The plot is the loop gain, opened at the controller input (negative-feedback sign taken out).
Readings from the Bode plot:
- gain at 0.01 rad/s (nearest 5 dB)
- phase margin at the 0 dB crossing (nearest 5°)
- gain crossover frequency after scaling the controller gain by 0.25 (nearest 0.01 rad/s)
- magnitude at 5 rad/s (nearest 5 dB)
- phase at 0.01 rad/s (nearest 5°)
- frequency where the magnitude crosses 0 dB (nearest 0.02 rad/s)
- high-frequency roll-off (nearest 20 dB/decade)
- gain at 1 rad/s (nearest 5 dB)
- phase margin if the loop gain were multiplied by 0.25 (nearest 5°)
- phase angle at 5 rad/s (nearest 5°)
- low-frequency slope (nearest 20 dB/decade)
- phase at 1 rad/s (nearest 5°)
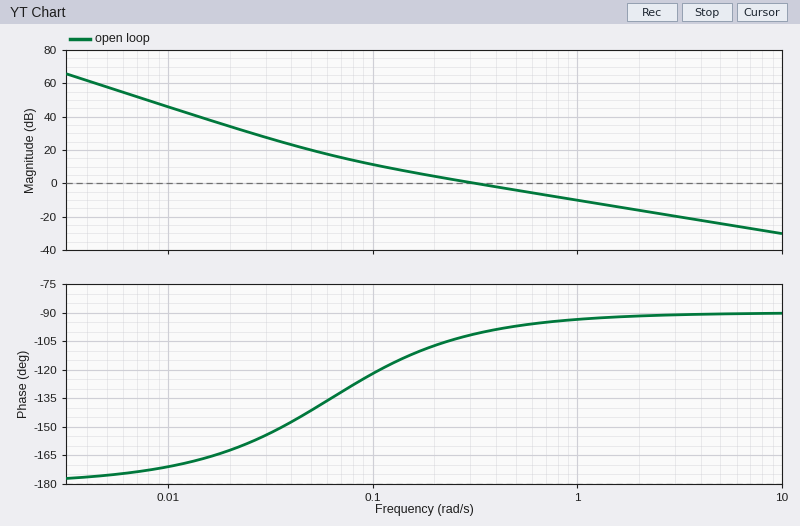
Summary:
45 dB
80°
0.09 rad/s
-25 dB
-170°
0.32 rad/s
-20 dB/decade
-10 dB
55°
-90°
-40 dB/decade
-95°
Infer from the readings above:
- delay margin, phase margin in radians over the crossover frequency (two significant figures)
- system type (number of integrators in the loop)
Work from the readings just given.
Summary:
4.4 s
2
